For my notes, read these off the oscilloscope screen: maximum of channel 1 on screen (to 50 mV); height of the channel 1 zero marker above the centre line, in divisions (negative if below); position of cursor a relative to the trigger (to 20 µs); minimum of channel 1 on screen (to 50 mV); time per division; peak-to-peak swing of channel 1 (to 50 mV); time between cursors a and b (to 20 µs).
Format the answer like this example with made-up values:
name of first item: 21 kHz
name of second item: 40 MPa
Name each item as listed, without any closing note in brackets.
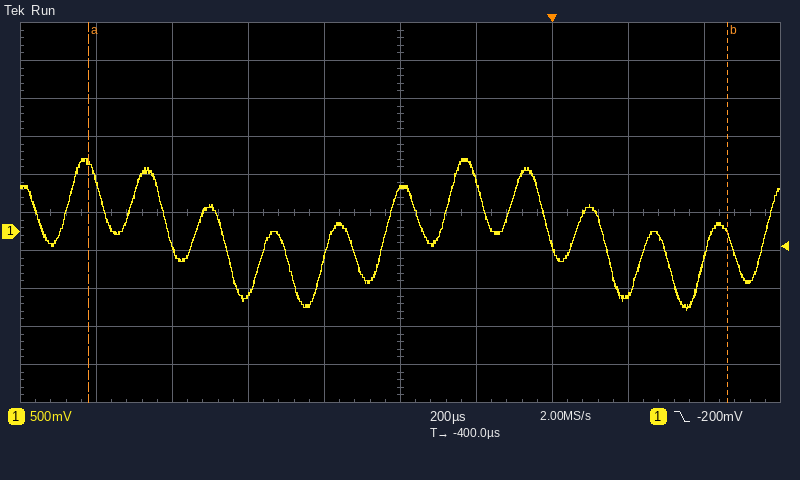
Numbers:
maximum of channel 1 on screen: 950 mV
height of the channel 1 zero marker above the centre line, in divisions: -0.5 div
position of cursor a relative to the trigger: -1.22 ms
minimum of channel 1 on screen: -1.05 V
time per division: 200 µs
peak-to-peak swing of channel 1: 2.00 V
time between cursors a and b: 1.68 ms
